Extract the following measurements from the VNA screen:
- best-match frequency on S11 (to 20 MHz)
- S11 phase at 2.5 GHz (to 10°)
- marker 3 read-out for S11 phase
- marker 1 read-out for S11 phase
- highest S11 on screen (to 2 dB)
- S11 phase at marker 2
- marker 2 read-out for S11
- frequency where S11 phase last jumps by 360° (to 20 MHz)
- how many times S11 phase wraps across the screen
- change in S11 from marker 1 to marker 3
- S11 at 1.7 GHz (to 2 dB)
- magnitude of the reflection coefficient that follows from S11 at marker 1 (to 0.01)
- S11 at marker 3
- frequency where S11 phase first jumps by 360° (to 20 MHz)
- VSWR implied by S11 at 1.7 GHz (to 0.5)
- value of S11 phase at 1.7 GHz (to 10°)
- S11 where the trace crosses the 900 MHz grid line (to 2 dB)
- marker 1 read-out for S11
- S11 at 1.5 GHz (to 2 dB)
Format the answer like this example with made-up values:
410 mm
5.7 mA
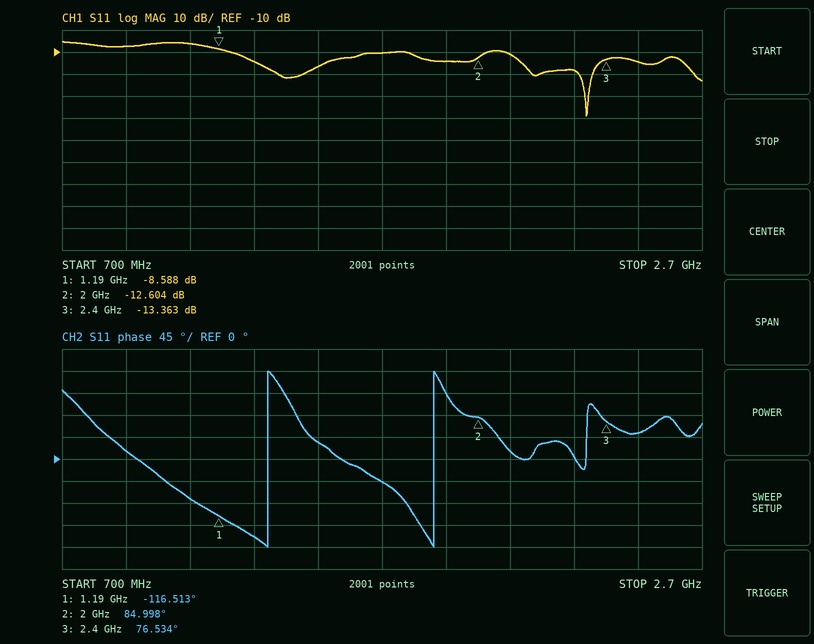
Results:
2.34 GHz
50°
76.534°
-116.513°
-6 dB
84.998°
-12.604 dB
1.86 GHz
2
-4.775 dB
-10 dB
0.37
-13.363 dB
1.34 GHz
2.0
-50°
-8 dB
-8.588 dB
-16 dB
